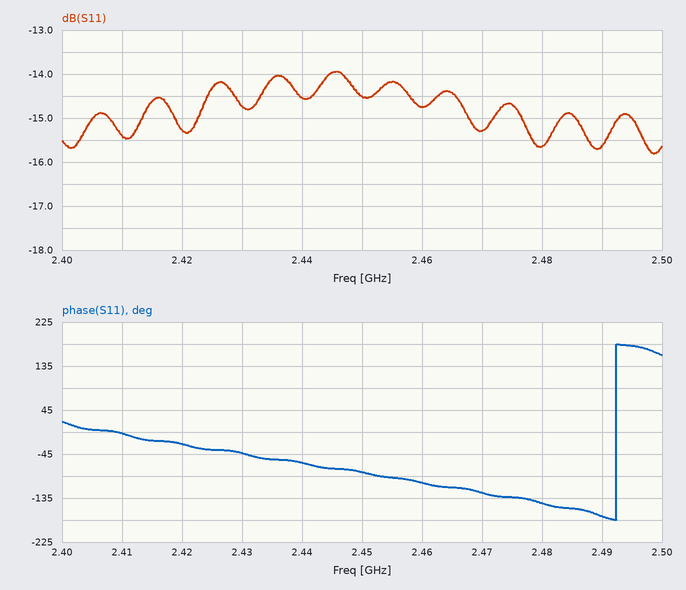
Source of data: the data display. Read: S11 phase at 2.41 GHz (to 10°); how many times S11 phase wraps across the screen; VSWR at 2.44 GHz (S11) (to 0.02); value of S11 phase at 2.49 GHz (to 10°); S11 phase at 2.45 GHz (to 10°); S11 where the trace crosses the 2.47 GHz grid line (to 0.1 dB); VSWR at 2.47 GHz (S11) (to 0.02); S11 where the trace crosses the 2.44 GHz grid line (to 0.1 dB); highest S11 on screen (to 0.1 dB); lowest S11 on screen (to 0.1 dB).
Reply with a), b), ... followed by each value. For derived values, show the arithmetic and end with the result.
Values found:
a) 0°
b) 1
c) |Γ| = 10^(-14.5/20) = 0.1884; VSWR = (1 + 0.1884)/(1 − 0.1884) ≈ 1.46
d) -170°
e) -80°
f) -15.3 dB
g) |Γ| = 10^(-15.3/20) = 0.1718; VSWR = (1 + 0.1718)/(1 − 0.1718) ≈ 1.41, so 1.42 to the nearest 0.02
h) -14.5 dB
i) -13.9 dB
j) -15.8 dB
